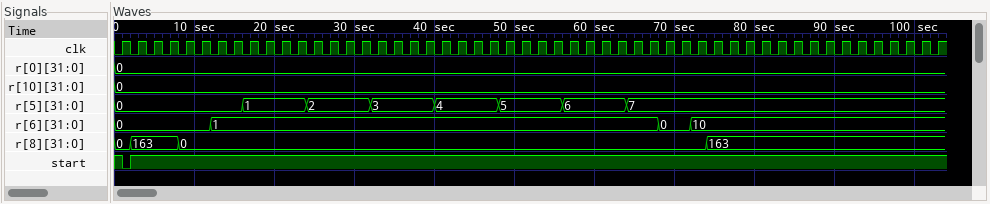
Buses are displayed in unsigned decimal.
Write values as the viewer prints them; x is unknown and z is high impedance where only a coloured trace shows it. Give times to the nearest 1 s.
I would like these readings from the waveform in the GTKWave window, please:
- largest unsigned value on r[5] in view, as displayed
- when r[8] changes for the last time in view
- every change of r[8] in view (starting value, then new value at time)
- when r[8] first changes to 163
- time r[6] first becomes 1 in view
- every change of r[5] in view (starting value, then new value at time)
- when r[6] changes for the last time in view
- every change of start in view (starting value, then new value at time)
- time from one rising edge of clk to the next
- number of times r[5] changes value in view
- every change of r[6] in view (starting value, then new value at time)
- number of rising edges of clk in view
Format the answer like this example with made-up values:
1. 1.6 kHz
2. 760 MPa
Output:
1. 7
2. 74 s
3. 0, 163 at 2 s, 0 at 8 s, 163 at 74 s
4. 2 s
5. 12 s
6. 0, 1 at 16 s, 2 at 24 s, 3 at 32 s, 4 at 40 s, 5 at 48 s, 6 at 56 s, 7 at 64 s
7. 72 s
8. 1, 0 at 1 s, 1 at 2 s
9. 2 s
10. 7
11. 0, 1 at 12 s, 0 at 68 s, 10 at 72 s
12. 52
